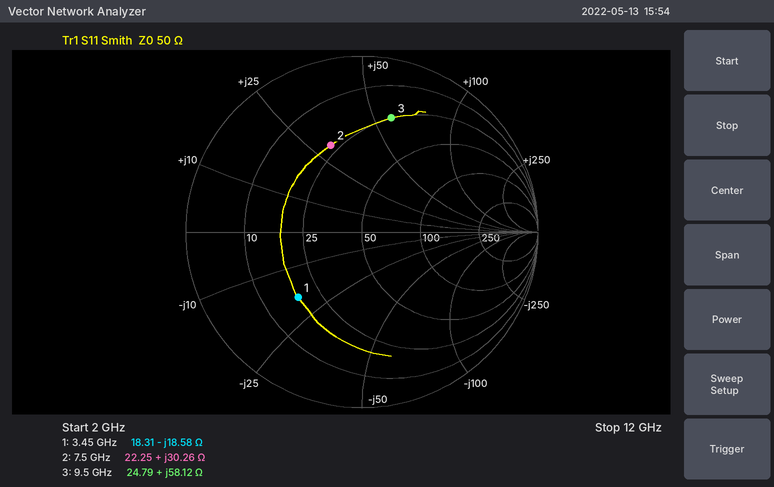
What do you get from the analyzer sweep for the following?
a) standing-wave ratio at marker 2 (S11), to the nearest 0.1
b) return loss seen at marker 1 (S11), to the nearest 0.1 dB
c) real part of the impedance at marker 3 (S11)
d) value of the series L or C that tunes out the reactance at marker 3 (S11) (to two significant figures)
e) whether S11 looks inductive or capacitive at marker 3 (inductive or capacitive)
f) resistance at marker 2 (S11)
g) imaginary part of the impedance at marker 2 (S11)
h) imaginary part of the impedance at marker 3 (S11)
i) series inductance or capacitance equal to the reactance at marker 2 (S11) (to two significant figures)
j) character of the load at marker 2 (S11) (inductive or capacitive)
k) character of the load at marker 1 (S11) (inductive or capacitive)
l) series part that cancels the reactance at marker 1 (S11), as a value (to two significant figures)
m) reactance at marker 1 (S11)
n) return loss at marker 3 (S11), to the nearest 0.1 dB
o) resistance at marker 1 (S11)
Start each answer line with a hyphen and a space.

- 3.2
- 5.7 dB
- 24.79 Ω
- 290 fF
- inductive
- 22.25 Ω
- +30.26 Ω
- +58.12 Ω
- 640 pH
- inductive
- capacitive
- 860 pH
- -18.58 Ω
- 3.5 dB
- 18.31 Ω
